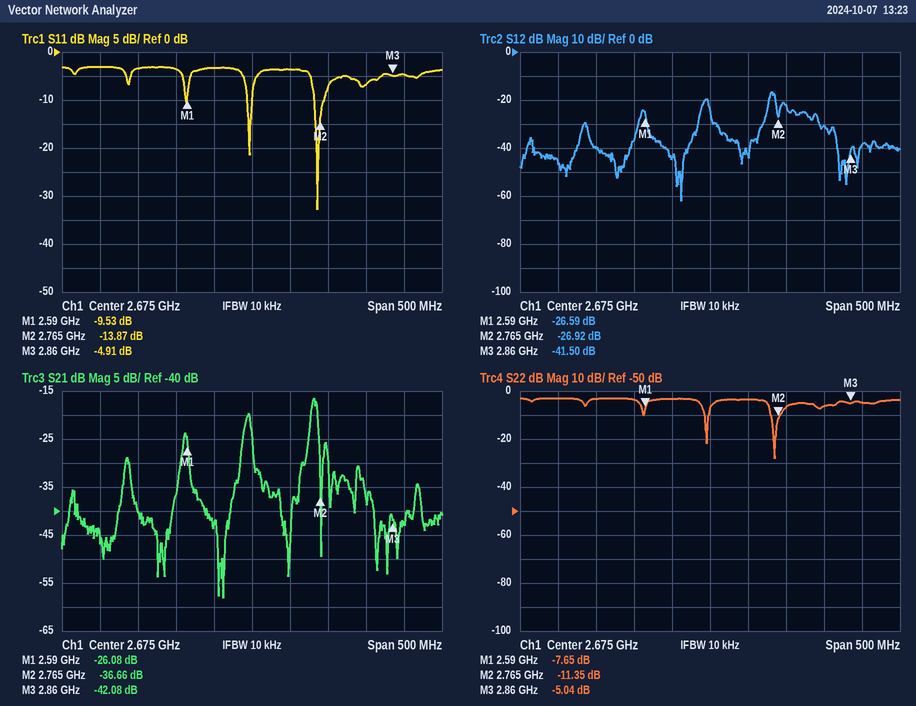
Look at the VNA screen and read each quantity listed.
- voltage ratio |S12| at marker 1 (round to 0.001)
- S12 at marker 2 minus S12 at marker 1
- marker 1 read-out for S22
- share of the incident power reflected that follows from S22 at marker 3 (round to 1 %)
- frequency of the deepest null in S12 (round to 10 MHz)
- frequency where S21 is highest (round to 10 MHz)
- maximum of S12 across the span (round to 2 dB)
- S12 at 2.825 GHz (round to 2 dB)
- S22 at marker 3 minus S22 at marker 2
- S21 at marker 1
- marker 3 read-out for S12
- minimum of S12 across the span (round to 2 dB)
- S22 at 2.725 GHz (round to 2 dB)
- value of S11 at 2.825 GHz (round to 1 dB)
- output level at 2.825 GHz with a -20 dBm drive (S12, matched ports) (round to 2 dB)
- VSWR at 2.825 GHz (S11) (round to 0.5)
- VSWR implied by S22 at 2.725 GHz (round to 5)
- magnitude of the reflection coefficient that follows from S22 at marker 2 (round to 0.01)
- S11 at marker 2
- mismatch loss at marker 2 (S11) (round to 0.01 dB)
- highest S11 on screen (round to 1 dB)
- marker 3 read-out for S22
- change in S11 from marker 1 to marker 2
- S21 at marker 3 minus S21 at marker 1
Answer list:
0.047
-0.33 dB
-7.65 dB
31 %
2.64 GHz
2.76 GHz
-16 dB
-30 dB
6.31 dB
-26.08 dB
-41.50 dB
-62 dB
-4 dB
-7 dB
-50 dBm
2.5
5
0.27
-13.87 dB
0.18 dB
-3 dB
-5.04 dB
-4.34 dB
-16.00 dB
